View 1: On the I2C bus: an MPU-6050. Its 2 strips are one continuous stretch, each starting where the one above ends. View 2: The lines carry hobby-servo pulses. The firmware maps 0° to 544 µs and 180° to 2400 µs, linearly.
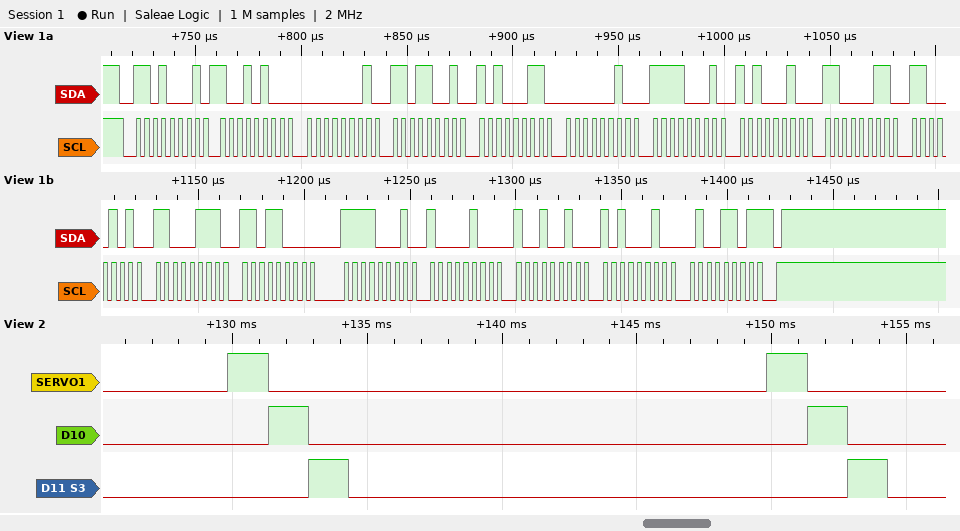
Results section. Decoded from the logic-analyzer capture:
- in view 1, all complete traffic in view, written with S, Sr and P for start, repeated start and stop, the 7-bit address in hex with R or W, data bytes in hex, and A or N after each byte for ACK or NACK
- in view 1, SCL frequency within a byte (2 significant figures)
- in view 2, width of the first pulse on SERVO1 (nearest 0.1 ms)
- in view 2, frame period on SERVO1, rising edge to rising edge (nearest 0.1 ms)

S 68R A 94 A 01 A D9 A A3 A 02 A F1 A A2 A C3 A C5 A C7 A D8 A F1 A 84 A 92 A A2 A 4D N P
250 kHz
1.5 ms
20.0 ms
